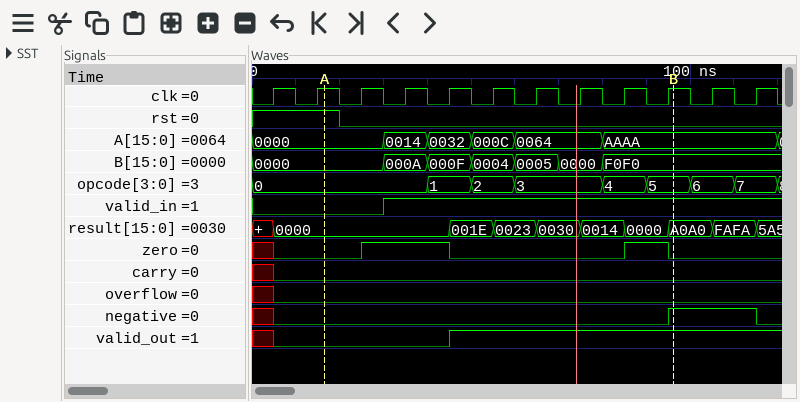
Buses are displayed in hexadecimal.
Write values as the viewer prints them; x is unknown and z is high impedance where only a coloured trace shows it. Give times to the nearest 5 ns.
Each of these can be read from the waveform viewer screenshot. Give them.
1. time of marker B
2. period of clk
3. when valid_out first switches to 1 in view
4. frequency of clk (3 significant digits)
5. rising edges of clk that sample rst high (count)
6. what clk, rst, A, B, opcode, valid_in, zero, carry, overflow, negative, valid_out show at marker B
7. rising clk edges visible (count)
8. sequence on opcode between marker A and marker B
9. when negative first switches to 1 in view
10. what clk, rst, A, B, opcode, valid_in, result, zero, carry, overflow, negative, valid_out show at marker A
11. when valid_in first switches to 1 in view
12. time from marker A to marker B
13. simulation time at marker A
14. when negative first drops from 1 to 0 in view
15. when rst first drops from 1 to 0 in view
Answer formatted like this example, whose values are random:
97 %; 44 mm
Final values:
95 ns; 10 ns; 45 ns; 100 MHz; 2; clk=1, rst=0, A=AAAA, B=F0F0, opcode=5, valid_in=1, zero=0, carry=0, overflow=0, negative=1, valid_out=1; 12; 0, 1, 2, 3, 4, 5; 95 ns; clk=1, rst=1, A=0000, B=0000, opcode=0, valid_in=0, result=0000, zero=0, carry=0, overflow=0, negative=0, valid_out=0; 30 ns; 80 ns; 15 ns; 115 ns; 20 ns
